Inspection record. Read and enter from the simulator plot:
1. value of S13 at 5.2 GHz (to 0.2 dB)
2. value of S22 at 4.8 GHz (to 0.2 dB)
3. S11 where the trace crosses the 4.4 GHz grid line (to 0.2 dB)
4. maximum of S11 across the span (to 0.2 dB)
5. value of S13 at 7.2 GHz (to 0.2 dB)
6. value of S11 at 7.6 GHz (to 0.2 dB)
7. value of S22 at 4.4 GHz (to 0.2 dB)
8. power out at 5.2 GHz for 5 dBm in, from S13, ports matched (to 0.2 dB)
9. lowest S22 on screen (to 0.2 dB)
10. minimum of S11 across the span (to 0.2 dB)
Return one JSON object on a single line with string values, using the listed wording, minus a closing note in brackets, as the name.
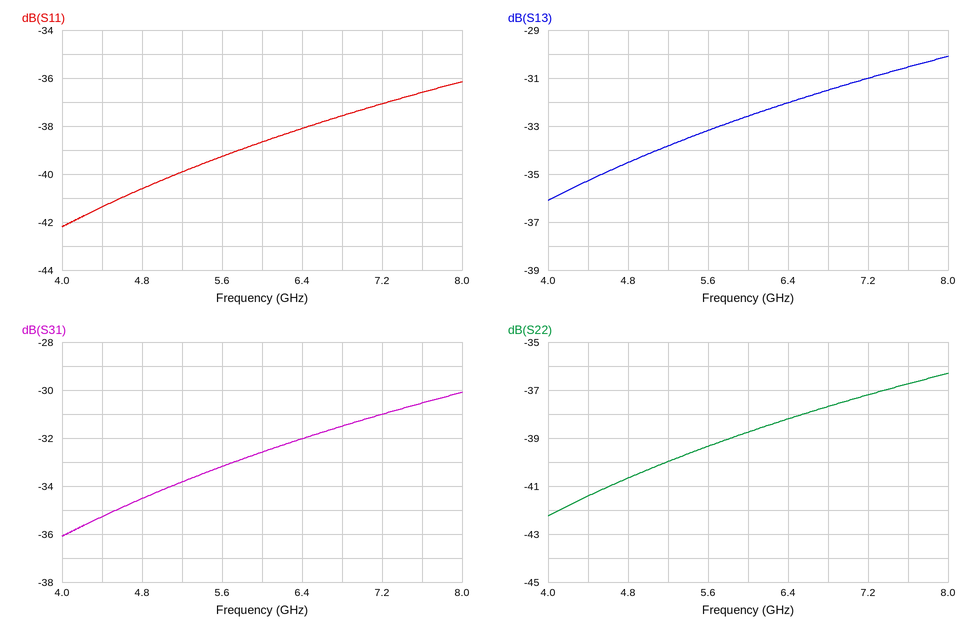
{"value of S13 at 5.2 GHz": "-33.8 dB", "value of S22 at 4.8 GHz": "-40.6 dB", "S11 where the trace crosses the 4.4 GHz grid line": "-41.4 dB", "maximum of S11 across the span": "-36.2 dB", "value of S13 at 7.2 GHz": "-31.0 dB", "value of S11 at 7.6 GHz": "-36.6 dB", "value of S22 at 4.4 GHz": "-41.4 dB", "power out at 5.2 GHz for 5 dBm in, from S13, ports matched": "-28.8 dBm", "lowest S22 on screen": "-42.2 dB", "minimum of S11 across the span": "-42.2 dB"}
